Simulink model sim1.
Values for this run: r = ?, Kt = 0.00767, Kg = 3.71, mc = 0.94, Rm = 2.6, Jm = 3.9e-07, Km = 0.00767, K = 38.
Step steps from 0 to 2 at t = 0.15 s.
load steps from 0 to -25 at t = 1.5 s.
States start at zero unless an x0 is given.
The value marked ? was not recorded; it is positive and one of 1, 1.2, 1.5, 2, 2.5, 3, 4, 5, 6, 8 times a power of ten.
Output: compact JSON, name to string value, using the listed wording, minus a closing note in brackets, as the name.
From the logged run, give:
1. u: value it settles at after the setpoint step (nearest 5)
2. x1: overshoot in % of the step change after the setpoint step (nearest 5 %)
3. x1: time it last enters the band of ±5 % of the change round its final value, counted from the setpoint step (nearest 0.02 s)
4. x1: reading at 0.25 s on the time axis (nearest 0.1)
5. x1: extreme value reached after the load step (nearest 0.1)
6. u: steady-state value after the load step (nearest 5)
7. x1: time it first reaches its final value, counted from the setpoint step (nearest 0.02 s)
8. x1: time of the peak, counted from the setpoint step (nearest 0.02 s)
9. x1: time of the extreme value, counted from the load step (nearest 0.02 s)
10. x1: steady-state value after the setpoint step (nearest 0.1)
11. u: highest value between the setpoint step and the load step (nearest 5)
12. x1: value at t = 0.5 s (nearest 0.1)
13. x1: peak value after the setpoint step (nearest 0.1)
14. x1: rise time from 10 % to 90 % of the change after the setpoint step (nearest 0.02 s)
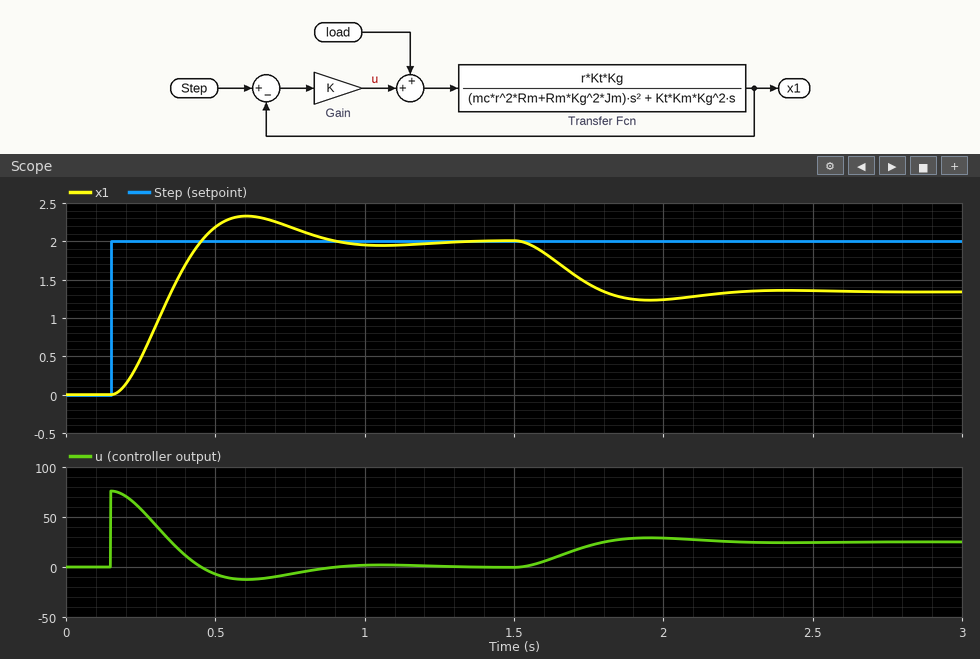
{"u: value it settles at after the setpoint step": "0", "x1: overshoot in % of the step change after the setpoint step": "15 %", "x1: time it last enters the band of ±5 % of the change round its final value, counted from the setpoint step": "0.66 s", "x1: reading at 0.25 s on the time axis": "0.5", "x1: extreme value reached after the load step": "1.2", "u: steady-state value after the load step": "25", "x1: time it first reaches its final value, counted from the setpoint step": "0.30 s", "x1: time of the peak, counted from the setpoint step": "0.46 s", "x1: time of the extreme value, counted from the load step": "0.46 s", "x1: steady-state value after the setpoint step": "2.0", "u: highest value between the setpoint step and the load step": "75", "x1: value at t = 0.5 s": "2.2", "x1: peak value after the setpoint step": "2.3", "x1: rise time from 10 % to 90 % of the change after the setpoint step": "0.20 s"}
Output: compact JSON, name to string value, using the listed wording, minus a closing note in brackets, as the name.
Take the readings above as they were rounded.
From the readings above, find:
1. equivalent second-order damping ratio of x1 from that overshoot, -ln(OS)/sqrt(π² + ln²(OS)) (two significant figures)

{"equivalent second-order damping ratio of x1 from that overshoot, -ln(OS)/sqrt(π² + ln²(OS))": "0.52"}
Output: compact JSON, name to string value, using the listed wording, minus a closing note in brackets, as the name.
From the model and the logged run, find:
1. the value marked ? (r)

{"the value marked ?": "0.006"}
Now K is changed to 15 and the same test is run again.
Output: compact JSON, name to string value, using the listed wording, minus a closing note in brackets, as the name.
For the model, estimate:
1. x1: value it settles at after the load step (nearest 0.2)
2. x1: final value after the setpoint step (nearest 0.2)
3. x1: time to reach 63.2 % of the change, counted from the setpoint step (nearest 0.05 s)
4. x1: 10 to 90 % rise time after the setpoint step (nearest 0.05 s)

{"x1: value it settles at after the load step": "0.4", "x1: final value after the setpoint step": "2.0", "x1: time to reach 63.2 % of the change, counted from the setpoint step": "0.35 s", "x1: 10 to 90 % rise time after the setpoint step": "0.50 s"}
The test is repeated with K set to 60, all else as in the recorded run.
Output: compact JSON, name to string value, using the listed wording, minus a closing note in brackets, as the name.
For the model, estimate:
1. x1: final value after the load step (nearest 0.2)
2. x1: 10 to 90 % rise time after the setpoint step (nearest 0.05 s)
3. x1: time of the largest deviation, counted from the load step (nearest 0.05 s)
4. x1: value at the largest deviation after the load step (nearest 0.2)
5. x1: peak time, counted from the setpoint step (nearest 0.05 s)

{"x1: final value after the load step": "1.6", "x1: 10 to 90 % rise time after the setpoint step": "0.15 s", "x1: time of the largest deviation, counted from the load step": "0.35 s", "x1: value at the largest deviation after the load step": "1.4", "x1: peak time, counted from the setpoint step": "0.35 s"}
